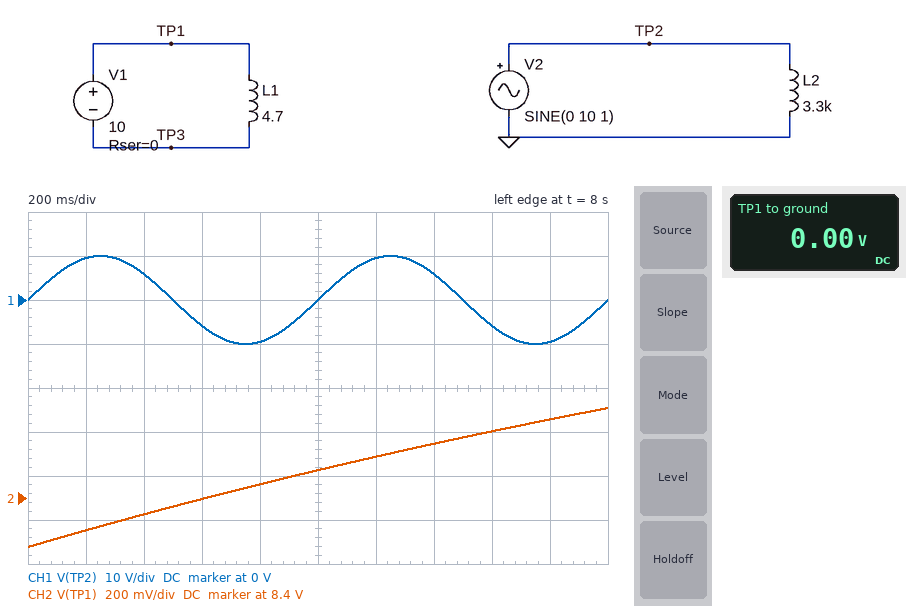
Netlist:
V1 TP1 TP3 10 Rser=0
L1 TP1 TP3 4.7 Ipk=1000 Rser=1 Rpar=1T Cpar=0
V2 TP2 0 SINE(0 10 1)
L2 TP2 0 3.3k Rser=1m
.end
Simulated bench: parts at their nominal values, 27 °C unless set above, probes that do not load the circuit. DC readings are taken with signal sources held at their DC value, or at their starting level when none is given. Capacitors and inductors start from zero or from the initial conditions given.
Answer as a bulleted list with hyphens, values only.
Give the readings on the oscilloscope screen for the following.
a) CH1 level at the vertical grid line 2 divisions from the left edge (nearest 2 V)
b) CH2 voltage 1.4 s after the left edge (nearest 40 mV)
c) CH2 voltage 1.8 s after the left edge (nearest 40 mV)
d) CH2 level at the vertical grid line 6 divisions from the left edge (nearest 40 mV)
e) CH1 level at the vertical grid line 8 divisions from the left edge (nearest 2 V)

- 6 V
- 8.64 V
- 8.76 V
- 8.60 V
- -6 V
